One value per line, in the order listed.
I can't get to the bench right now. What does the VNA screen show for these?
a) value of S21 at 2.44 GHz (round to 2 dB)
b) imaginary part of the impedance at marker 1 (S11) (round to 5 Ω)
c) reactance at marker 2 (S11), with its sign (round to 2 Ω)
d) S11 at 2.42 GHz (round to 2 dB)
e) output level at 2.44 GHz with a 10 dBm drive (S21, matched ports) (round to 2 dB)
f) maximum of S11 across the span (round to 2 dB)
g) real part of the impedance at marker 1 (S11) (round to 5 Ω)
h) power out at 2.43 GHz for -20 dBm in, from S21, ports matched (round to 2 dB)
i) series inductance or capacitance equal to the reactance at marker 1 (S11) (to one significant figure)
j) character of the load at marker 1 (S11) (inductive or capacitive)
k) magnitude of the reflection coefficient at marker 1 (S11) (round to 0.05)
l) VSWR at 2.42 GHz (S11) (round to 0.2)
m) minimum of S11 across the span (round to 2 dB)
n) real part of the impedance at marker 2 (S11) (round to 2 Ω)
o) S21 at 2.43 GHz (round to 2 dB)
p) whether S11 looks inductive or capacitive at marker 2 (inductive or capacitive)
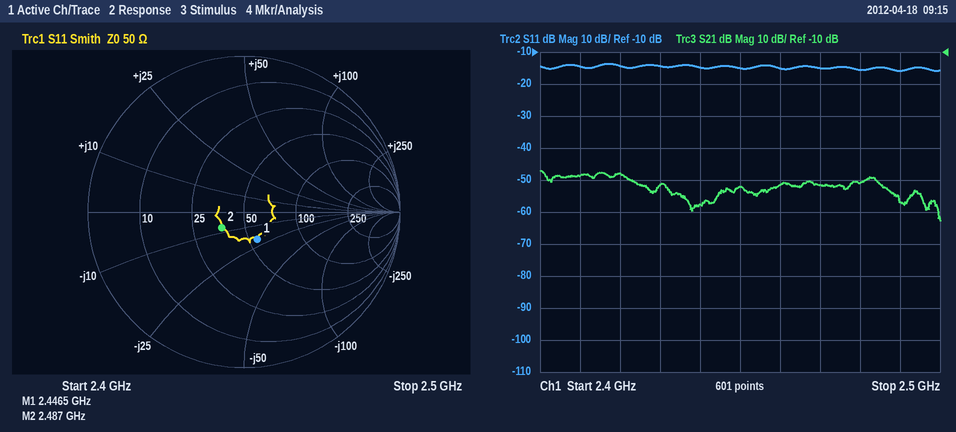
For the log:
-58 dB
-20 Ω
-8 Ω
-14 dB
-48 dBm
-14 dB
55 Ω
-72 dBm
3 pF
capacitive
0.20
1.4
-16 dB
36 Ω
-52 dB
capacitive
